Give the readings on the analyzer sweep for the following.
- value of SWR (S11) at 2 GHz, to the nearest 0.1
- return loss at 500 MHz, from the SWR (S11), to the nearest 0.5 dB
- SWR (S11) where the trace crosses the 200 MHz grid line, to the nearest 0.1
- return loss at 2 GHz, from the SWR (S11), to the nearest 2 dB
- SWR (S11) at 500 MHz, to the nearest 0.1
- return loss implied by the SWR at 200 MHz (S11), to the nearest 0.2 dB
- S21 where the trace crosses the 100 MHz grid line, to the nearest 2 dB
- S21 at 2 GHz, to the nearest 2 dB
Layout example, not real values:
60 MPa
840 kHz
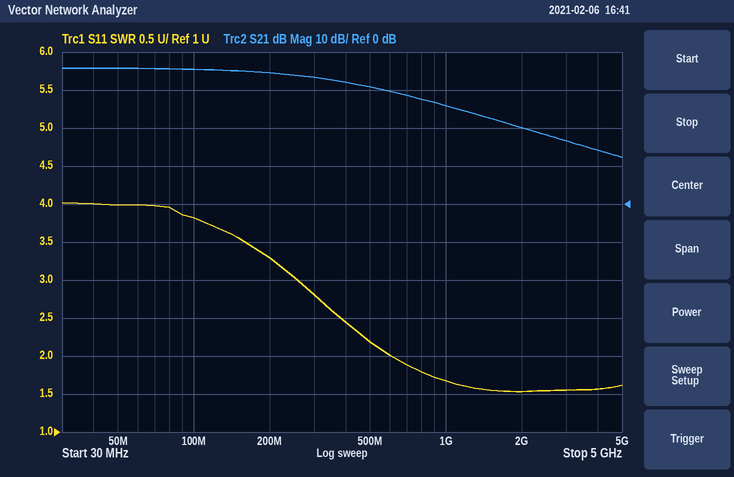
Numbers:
1.5
8.5 dB
3.3
14 dB
2.2
5.4 dB
36 dB
20 dB
